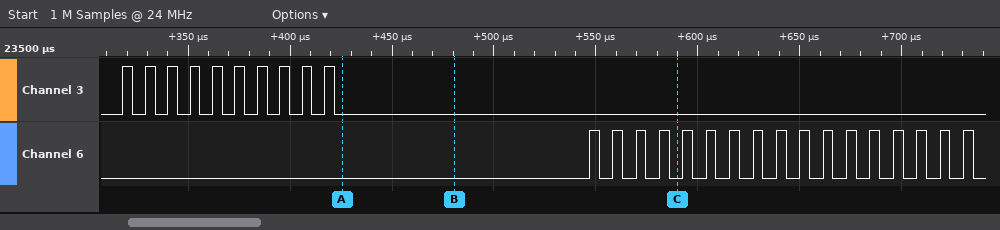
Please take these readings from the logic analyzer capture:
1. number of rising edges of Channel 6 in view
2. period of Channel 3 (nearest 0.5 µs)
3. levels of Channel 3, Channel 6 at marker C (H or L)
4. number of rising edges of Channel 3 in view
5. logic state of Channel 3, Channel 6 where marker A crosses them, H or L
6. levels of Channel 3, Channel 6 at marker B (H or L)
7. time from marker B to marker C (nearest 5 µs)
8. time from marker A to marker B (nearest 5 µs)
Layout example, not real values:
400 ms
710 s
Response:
17
11 µs
Channel 3=L, Channel 6=L
10
Channel 3=L, Channel 6=L
Channel 3=L, Channel 6=L
110 µs
55 µs
